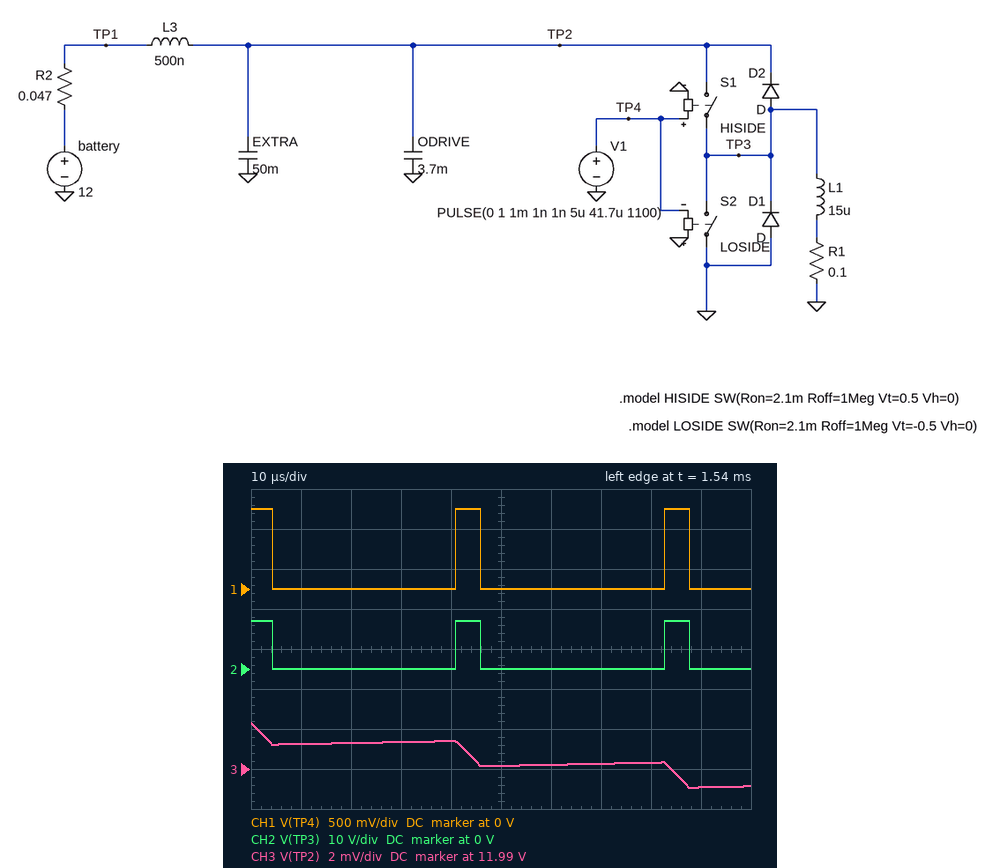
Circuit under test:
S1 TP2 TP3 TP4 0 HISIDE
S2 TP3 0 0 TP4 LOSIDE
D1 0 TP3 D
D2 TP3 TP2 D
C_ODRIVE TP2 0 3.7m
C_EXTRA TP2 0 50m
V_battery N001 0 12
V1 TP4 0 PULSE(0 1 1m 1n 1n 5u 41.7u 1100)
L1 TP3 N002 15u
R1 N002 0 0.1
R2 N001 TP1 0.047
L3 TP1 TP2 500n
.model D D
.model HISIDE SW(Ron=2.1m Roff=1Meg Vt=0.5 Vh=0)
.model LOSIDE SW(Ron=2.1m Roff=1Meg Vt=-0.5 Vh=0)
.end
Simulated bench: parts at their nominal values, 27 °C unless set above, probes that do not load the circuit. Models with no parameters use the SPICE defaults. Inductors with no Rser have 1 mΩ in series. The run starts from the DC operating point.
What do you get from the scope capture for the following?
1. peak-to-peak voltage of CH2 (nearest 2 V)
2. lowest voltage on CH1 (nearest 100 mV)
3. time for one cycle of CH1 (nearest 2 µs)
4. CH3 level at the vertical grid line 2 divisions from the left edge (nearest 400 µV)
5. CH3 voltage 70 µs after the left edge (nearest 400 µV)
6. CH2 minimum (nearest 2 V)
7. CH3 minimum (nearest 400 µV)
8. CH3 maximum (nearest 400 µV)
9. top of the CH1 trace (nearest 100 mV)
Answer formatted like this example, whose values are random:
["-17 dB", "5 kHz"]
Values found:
["12 V", "0 V", "42 µs", "11.9872 V", "11.9864 V", "0 V", "11.9852 V", "11.9884 V", "1.0 V"]
